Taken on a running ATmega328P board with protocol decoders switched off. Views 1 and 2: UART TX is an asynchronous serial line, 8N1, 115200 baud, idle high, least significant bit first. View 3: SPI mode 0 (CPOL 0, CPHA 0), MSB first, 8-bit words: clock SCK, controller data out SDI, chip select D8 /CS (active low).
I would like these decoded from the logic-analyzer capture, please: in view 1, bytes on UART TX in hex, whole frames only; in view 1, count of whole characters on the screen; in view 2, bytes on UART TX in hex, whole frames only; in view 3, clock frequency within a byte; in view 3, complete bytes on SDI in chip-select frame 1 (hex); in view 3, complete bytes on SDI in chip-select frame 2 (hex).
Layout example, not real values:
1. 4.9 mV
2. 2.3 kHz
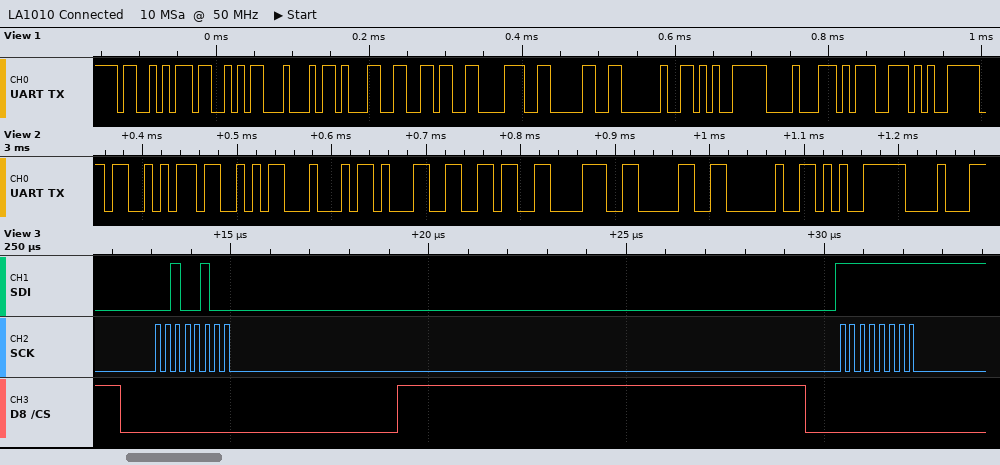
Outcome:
1. 53 53 44 31 36 38 30 20 E5 88 9D E5
2. 12
3. 53 53 44 31 36 38 30 20 E5 88
4. 4 MHz
5. 0x24
6. 0xFF
